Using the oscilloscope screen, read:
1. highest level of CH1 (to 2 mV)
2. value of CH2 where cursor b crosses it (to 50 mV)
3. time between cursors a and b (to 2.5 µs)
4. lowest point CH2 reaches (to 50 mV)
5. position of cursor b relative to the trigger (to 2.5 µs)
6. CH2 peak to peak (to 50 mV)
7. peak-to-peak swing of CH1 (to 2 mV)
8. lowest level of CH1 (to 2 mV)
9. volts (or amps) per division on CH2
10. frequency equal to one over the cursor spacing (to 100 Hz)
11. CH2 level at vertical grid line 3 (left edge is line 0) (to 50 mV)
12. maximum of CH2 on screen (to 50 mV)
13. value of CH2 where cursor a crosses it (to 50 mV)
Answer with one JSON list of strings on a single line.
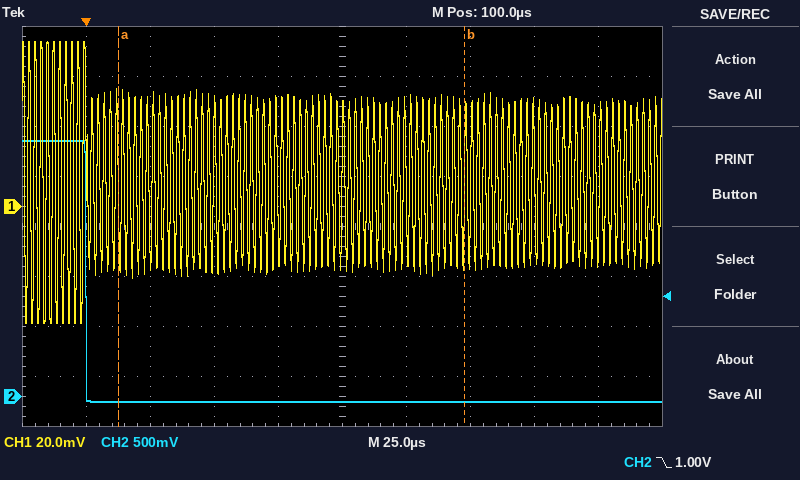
["66 mV", "-50 mV", "135.0 µs", "-50 mV", "+147.5 µs", "2.60 V", "112 mV", "-46 mV", "500 mV", "7.4 kHz", "-50 mV", "2.55 V", "-50 mV"]
